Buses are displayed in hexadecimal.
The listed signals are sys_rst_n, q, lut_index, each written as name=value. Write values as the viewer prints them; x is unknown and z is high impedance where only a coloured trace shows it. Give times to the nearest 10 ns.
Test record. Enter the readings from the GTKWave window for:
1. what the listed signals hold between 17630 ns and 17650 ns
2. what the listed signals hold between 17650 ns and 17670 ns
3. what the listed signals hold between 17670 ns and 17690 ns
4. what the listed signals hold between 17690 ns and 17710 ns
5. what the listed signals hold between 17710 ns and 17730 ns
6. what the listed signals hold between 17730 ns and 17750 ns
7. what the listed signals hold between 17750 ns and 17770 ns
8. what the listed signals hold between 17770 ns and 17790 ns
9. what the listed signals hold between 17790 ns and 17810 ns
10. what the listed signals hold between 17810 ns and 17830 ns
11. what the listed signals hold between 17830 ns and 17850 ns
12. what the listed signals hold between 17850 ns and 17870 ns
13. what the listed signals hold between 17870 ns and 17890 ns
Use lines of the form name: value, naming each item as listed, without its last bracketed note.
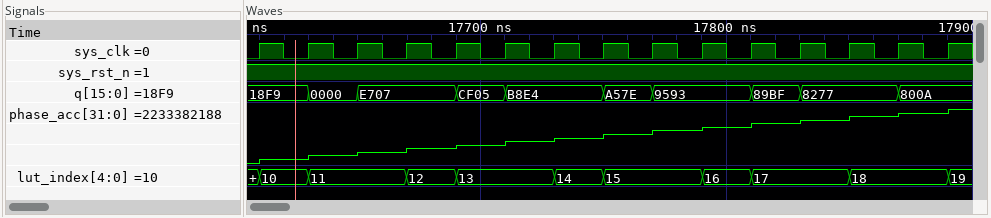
what the listed signals hold between 17630 ns and 17650 ns: sys_rst_n=1, q=0000, lut_index=11
what the listed signals hold between 17650 ns and 17670 ns: sys_rst_n=1, q=E707, lut_index=11
what the listed signals hold between 17670 ns and 17690 ns: sys_rst_n=1, q=E707, lut_index=12
what the listed signals hold between 17690 ns and 17710 ns: sys_rst_n=1, q=CF05, lut_index=13
what the listed signals hold between 17710 ns and 17730 ns: sys_rst_n=1, q=B8E4, lut_index=13
what the listed signals hold between 17730 ns and 17750 ns: sys_rst_n=1, q=B8E4, lut_index=14
what the listed signals hold between 17750 ns and 17770 ns: sys_rst_n=1, q=A57E, lut_index=15
what the listed signals hold between 17770 ns and 17790 ns: sys_rst_n=1, q=9593, lut_index=15
what the listed signals hold between 17790 ns and 17810 ns: sys_rst_n=1, q=9593, lut_index=16
what the listed signals hold between 17810 ns and 17830 ns: sys_rst_n=1, q=89BF, lut_index=17
what the listed signals hold between 17830 ns and 17850 ns: sys_rst_n=1, q=8277, lut_index=17
what the listed signals hold between 17850 ns and 17870 ns: sys_rst_n=1, q=8277, lut_index=18
what the listed signals hold between 17870 ns and 17890 ns: sys_rst_n=1, q=800A, lut_index=18
